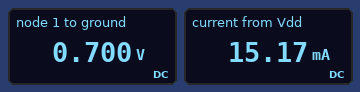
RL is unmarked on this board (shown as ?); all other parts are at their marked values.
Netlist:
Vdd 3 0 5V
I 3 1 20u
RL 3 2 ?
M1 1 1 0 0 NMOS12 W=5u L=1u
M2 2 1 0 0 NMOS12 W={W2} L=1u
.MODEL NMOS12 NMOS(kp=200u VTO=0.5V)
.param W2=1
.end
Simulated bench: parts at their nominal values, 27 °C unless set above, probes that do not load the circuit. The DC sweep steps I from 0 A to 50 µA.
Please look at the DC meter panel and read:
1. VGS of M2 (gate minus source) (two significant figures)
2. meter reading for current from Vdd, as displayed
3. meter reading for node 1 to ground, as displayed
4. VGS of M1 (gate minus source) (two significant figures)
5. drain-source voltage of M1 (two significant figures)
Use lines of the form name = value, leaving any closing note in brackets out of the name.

VGS of M2 (gate minus source) = 700 mV
meter reading for current from Vdd, as displayed = 15.17 mA
meter reading for node 1 to ground, as displayed = 0.700 V
VGS of M1 (gate minus source) = 700 mV
drain-source voltage of M1 = 700 mV
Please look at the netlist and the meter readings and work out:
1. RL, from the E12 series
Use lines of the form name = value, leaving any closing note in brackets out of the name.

RL, from the E12 series = 330 Ω
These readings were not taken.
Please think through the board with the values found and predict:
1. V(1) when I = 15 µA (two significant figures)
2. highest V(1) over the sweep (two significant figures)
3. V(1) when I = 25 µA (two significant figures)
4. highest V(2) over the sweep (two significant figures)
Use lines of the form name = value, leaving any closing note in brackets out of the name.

V(1) when I = 15 µA = 670 mV
highest V(1) over the sweep = 820 mV
V(1) when I = 25 µA = 720 mV
highest V(2) over the sweep = 5.0 V
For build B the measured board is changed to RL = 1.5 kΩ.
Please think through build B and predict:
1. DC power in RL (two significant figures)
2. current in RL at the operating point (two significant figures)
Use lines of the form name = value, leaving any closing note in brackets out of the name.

DC power in RL = 17 mW
current in RL at the operating point = 3.3 mA
